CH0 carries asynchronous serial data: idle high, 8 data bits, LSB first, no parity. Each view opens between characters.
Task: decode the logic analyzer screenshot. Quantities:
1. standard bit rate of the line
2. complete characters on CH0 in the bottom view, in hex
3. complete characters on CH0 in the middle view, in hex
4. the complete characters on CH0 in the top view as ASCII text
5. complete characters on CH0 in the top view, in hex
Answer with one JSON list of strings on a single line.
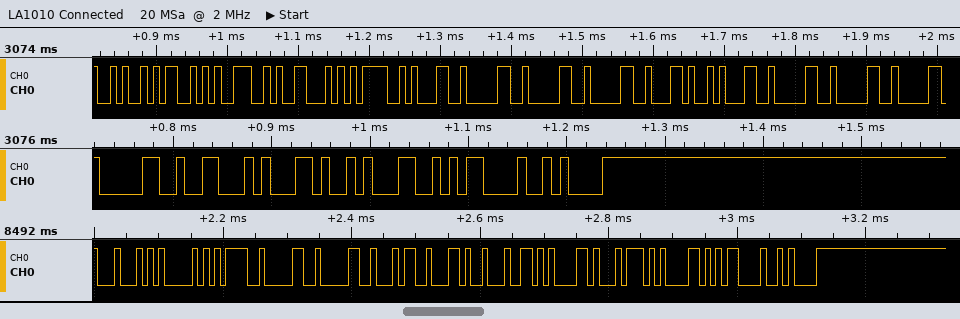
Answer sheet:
["115200 baud", "44, 41, 3D, 30, 30, 34, 2C, 64, 61, 74, 61, 0D, 0A", "30, 46, 2C, 31, 0D, 0A", "\"JSNF=1000,100\"", "4A, 53, 4E, 46, 3D, 31, 30, 30, 30, 2C, 31, 30, 30"]
